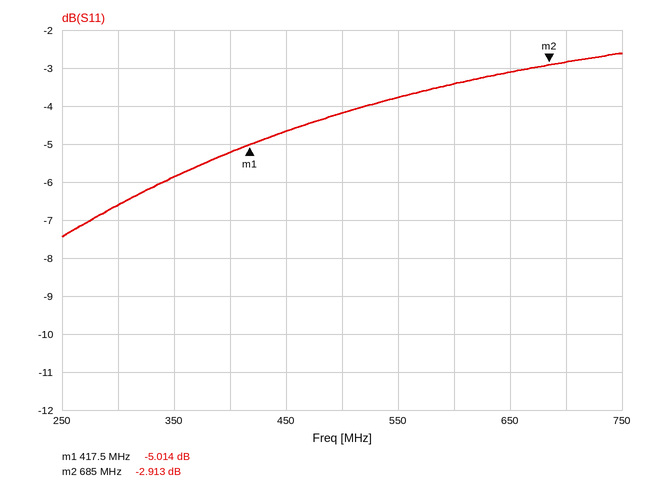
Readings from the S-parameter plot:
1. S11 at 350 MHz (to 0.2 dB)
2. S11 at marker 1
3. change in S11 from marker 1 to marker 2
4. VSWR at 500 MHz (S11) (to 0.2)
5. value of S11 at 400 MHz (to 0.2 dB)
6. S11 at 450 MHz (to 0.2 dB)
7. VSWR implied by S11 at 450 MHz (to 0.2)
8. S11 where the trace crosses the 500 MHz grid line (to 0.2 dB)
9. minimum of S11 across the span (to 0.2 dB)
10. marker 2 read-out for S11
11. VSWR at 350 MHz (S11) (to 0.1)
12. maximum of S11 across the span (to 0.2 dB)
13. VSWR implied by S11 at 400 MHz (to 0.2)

-5.8 dB
-5.014 dB
2.101 dB
4.2
-5.2 dB
-4.6 dB
3.8
-4.2 dB
-7.4 dB
-2.913 dB
3.1
-2.6 dB
3.4
